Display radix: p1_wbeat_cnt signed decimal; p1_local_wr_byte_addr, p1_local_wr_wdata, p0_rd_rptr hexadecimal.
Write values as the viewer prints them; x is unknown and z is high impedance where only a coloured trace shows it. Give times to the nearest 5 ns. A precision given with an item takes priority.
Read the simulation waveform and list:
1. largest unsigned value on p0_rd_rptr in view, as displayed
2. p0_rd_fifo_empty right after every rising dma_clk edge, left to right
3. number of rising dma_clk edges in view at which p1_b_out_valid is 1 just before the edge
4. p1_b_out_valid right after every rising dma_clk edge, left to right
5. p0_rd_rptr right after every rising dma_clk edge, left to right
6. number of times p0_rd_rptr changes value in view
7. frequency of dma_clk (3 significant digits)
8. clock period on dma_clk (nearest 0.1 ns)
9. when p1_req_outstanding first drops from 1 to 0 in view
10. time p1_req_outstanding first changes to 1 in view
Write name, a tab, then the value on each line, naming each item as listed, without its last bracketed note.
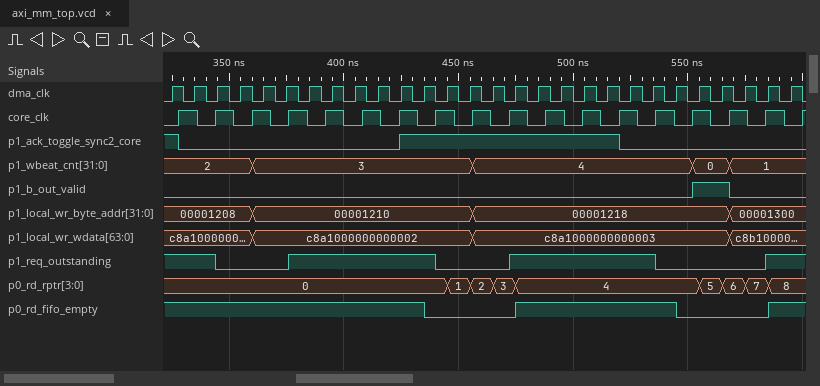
largest unsigned value on p0_rd_rptr in view, as displayed	8
p0_rd_fifo_empty right after every rising dma_clk edge, left to right	1 1 1 1 1 1 1 1 1 1 1 0 0 0 0 1 1 1 1 1 1 1 0 0 0 0 1 1
number of rising dma_clk edges in view at which p1_b_out_valid is 1 just before the edge	2
p1_b_out_valid right after every rising dma_clk edge, left to right	0 0 0 0 0 0 0 0 0 0 0 0 0 0 0 0 0 0 0 0 0 0 0 1 1 0 0 0
p0_rd_rptr right after every rising dma_clk edge, left to right	0, 0, 0, 0, 0, 0, 0, 0, 0, 0, 0, 0, 1, 2, 3, 4, 4, 4, 4, 4, 4, 4, 4, 5, 6, 7, 8, 8
number of times p0_rd_rptr changes value in view	8
frequency of dma_clk	100 MHz
clock period on dma_clk	10 ns
when p1_req_outstanding first drops from 1 to 0 in view	345 ns
time p1_req_outstanding first changes to 1 in view	375 ns
